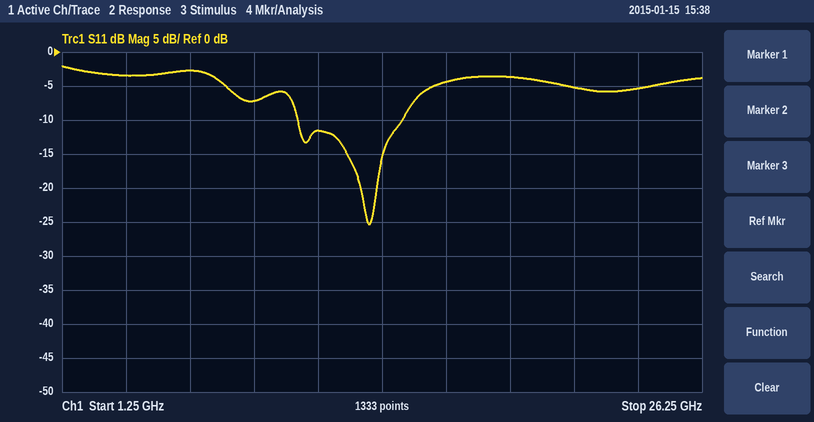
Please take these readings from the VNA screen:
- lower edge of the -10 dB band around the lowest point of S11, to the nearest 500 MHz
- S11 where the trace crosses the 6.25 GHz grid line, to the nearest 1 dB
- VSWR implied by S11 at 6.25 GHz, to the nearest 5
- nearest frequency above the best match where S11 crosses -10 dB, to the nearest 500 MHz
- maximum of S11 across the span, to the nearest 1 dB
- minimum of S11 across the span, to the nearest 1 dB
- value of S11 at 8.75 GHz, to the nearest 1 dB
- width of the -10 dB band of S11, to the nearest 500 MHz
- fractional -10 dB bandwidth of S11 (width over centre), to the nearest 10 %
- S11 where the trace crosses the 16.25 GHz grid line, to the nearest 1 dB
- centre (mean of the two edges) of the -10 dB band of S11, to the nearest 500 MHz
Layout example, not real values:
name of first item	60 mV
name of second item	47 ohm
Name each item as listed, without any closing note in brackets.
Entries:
lower edge of the -10 dB band around the lowest point of S11, to the nearest 500 MHz	10.5 GHz
S11 where the trace crosses the 6.25 GHz grid line, to the nearest 1 dB	-3 dB
VSWR implied by S11 at 6.25 GHz, to the nearest 5	5
nearest frequency above the best match where S11 crosses -10 dB, to the nearest 500 MHz	14.5 GHz
maximum of S11 across the span, to the nearest 1 dB	-2 dB
minimum of S11 across the span, to the nearest 1 dB	-25 dB
value of S11 at 8.75 GHz, to the nearest 1 dB	-7 dB
width of the -10 dB band of S11, to the nearest 500 MHz	4.0 GHz
fractional -10 dB bandwidth of S11 (width over centre), to the nearest 10 %	30 %
S11 where the trace crosses the 16.25 GHz grid line, to the nearest 1 dB	-4 dB
centre (mean of the two edges) of the -10 dB band of S11, to the nearest 500 MHz	12.5 GHz
